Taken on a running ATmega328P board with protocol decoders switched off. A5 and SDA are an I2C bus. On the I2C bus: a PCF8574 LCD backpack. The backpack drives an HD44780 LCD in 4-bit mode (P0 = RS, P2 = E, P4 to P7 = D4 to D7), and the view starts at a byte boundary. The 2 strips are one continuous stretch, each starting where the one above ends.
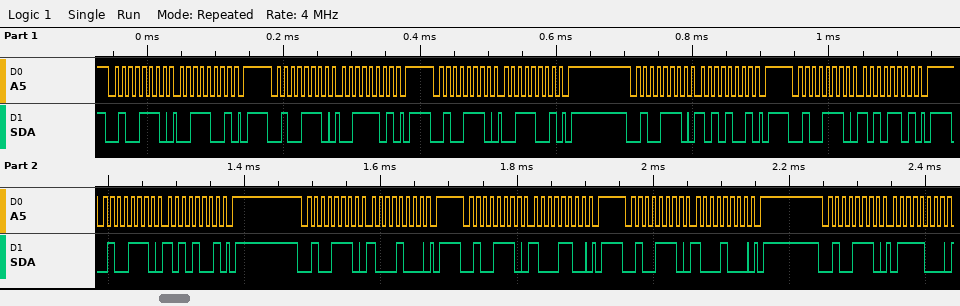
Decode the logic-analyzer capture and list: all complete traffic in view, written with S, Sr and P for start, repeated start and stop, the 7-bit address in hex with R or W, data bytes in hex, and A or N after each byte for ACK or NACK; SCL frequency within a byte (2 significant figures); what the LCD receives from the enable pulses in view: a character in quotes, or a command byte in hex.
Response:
S 27W A 39 A P S 27W A 3D A P S 27W A 39 A P S 27W A A9 A P S 27W A AD A P S 27W A A9 A P S 27W A 88 A P S 27W A 8C A P S 27W A 88 A P S 27W A 78 A
100 kHz
':'
